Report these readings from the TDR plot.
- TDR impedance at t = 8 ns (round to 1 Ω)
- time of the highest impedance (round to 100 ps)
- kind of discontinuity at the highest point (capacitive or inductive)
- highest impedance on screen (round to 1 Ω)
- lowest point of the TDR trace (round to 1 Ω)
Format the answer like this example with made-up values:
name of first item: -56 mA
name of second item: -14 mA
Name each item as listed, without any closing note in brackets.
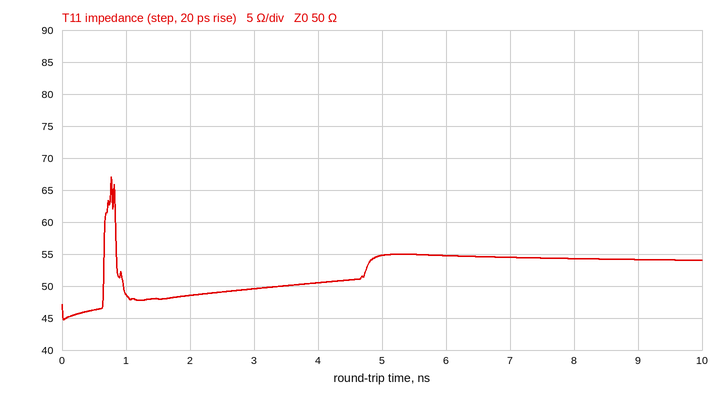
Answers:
TDR impedance at t = 8 ns: 54 Ω
time of the highest impedance: 800 ps
kind of discontinuity at the highest point: inductive
highest impedance on screen: 67 Ω
lowest point of the TDR trace: 45 Ω
